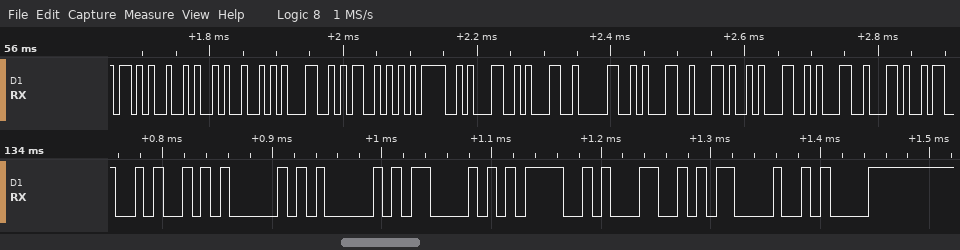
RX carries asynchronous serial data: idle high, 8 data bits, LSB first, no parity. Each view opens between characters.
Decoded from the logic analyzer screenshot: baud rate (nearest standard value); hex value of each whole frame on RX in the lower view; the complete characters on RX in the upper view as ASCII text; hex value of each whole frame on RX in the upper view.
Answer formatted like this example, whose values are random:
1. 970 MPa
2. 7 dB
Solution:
1. 115200 baud
2. 4A, 41, 41, 43, 3D, 31, 0D, 0A
3. "+JRLS=1101,11,"
4. 2B, 4A, 52, 4C, 53, 3D, 31, 31, 30, 31, 2C, 31, 31, 2C
